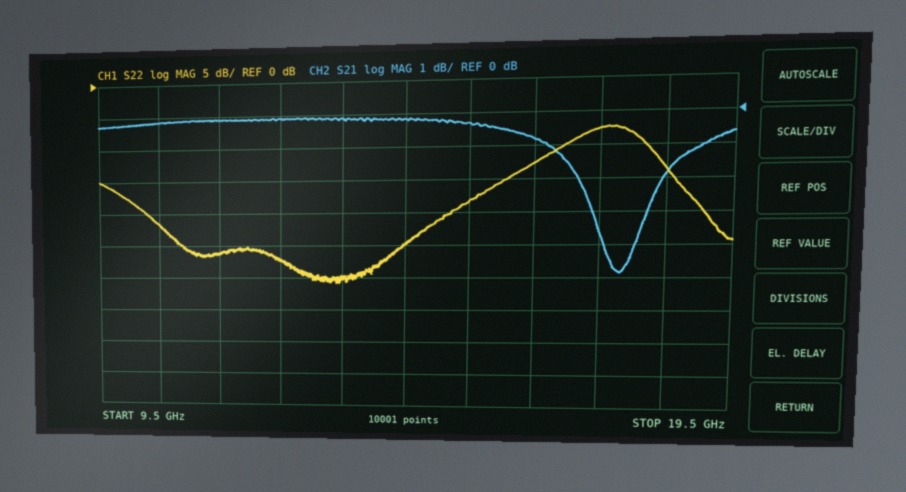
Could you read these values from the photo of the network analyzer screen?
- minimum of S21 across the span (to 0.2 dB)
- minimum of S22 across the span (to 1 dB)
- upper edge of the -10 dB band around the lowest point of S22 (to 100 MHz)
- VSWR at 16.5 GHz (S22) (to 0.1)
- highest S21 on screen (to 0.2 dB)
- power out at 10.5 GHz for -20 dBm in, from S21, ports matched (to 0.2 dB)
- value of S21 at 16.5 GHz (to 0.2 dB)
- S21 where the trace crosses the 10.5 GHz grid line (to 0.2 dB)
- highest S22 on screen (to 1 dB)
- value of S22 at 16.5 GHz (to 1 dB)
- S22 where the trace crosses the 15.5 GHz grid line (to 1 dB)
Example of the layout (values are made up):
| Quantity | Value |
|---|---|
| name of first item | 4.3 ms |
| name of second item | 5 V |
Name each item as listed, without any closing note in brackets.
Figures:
| Quantity | Value |
|---|---|
| minimum of S21 across the span | -4.8 dB |
| minimum of S22 across the span | -31 dB |
| upper edge of the -10 dB band around the lowest point of S22 | 17.0 GHz |
| VSWR at 16.5 GHz (S22) | 1.6 |
| highest S21 on screen | 0.0 dB |
| power out at 10.5 GHz for -20 dBm in, from S21, ports matched | -20.2 dBm |
| value of S21 at 16.5 GHz | -0.8 dB |
| S21 where the trace crosses the 10.5 GHz grid line | -0.2 dB |
| highest S22 on screen | -7 dB |
| value of S22 at 16.5 GHz | -13 dB |
| S22 where the trace crosses the 15.5 GHz grid line | -18 dB |
